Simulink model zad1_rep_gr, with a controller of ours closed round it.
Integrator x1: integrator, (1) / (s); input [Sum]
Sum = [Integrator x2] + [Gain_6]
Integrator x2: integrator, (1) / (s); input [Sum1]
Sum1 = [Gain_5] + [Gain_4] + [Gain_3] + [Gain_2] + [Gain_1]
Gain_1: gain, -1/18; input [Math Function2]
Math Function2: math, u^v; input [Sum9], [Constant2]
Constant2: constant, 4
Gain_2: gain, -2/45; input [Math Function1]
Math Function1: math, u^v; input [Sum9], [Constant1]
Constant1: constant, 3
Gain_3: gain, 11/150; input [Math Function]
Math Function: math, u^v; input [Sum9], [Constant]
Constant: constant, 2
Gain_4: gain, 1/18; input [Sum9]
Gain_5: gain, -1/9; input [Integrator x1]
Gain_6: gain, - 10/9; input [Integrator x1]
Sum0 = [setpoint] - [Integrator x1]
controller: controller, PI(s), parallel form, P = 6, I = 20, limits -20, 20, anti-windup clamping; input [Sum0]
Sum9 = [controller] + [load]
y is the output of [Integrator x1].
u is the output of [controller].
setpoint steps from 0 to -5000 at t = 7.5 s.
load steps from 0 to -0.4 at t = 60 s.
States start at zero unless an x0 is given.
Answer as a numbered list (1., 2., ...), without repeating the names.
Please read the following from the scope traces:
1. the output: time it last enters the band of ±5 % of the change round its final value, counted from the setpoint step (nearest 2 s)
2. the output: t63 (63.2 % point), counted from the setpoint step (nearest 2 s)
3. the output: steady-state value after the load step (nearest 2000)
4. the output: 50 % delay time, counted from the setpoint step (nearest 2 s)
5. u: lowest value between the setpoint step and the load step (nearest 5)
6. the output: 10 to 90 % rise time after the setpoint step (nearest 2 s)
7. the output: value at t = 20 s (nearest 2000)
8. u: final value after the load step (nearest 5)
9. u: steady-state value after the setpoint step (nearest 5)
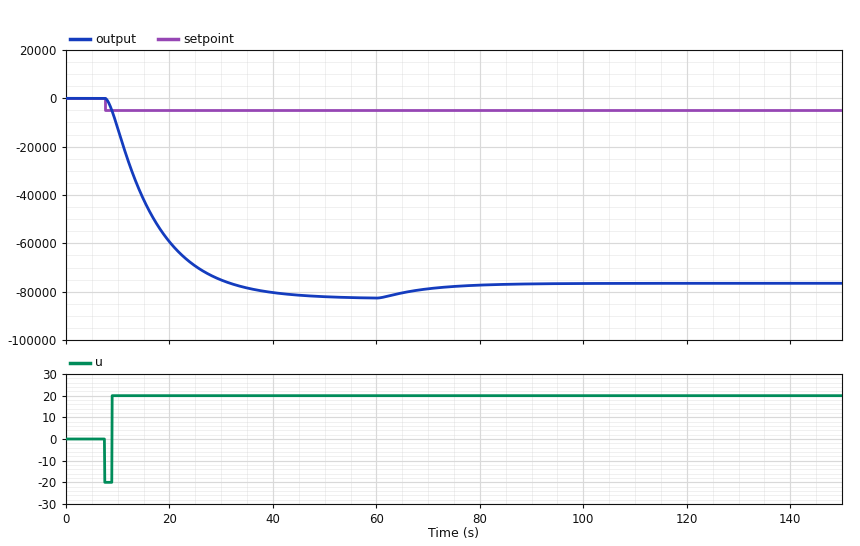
1. 28 s
2. 10 s
3. -76000
4. 8 s
5. -20
6. 20 s
7. -60000
8. 20
9. 20
